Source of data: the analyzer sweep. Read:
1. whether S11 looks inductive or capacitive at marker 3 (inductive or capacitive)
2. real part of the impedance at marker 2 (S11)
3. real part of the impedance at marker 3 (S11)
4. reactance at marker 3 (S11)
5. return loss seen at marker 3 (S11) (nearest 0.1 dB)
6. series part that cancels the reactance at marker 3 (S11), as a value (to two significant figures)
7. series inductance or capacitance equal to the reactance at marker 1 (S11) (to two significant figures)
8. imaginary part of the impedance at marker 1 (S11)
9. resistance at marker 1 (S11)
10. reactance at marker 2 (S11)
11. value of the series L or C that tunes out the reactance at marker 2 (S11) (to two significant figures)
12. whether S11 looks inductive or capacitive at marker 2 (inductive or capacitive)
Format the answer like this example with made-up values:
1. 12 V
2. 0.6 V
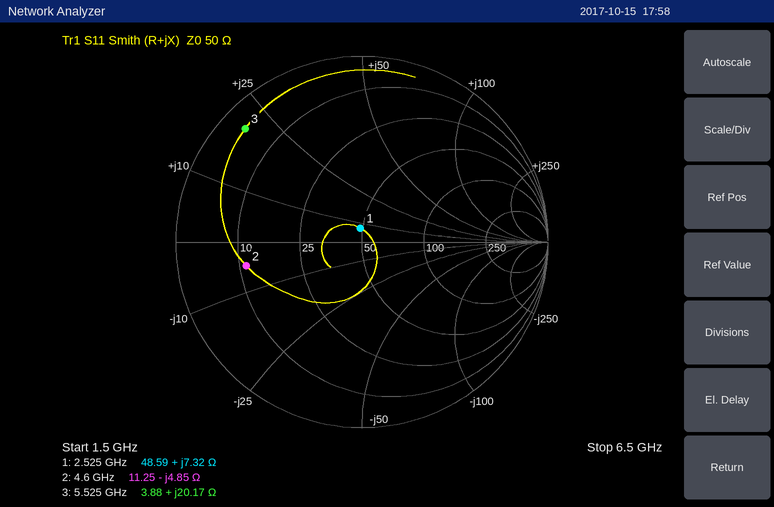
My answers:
1. inductive
2. 11.25 Ω
3. 3.88 Ω
4. +20.17 Ω
5. 1.2 dB
6. 1.4 pF
7. 460 pH
8. +7.32 Ω
9. 48.59 Ω
10. -4.85 Ω
11. 170 pH
12. capacitive
